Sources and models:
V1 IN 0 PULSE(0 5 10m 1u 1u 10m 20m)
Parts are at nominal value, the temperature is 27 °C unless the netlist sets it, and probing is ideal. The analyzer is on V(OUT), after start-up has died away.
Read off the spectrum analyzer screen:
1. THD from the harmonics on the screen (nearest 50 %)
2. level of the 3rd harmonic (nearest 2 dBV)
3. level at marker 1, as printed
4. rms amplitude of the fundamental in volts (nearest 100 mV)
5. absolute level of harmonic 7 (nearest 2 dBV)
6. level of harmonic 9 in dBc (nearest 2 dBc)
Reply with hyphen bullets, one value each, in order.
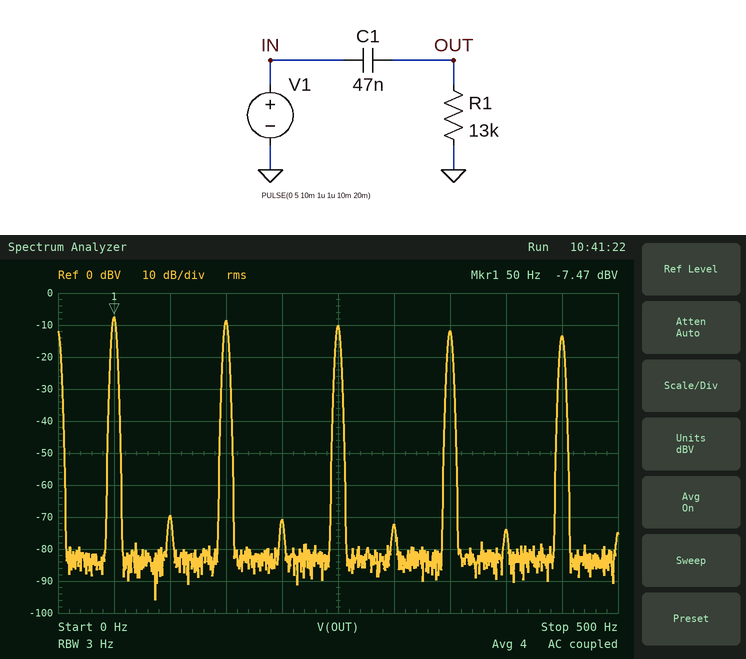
- 150 %
- -8 dBV
- -7.47 dBV
- 400 mV
- -12 dBV
- -6 dBc
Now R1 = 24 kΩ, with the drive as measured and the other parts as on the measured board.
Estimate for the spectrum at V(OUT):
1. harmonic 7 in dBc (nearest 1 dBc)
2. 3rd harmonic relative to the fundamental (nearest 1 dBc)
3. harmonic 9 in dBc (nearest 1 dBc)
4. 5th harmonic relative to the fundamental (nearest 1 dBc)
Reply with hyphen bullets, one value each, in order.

- -8 dBc
- -3 dBc
- -10 dBc
- -6 dBc
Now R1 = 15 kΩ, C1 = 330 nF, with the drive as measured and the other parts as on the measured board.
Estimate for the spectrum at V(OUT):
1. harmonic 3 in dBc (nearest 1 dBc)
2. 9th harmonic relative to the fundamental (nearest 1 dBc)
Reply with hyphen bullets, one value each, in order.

- -8 dBc
- -18 dBc
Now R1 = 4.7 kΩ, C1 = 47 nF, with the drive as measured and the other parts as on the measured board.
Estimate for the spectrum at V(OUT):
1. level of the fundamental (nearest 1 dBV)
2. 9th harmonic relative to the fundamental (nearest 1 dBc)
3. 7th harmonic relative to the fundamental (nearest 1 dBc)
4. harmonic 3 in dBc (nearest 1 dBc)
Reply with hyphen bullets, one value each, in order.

- -16 dBV
- -1 dBc
- -1 dBc
- 0 dBc
